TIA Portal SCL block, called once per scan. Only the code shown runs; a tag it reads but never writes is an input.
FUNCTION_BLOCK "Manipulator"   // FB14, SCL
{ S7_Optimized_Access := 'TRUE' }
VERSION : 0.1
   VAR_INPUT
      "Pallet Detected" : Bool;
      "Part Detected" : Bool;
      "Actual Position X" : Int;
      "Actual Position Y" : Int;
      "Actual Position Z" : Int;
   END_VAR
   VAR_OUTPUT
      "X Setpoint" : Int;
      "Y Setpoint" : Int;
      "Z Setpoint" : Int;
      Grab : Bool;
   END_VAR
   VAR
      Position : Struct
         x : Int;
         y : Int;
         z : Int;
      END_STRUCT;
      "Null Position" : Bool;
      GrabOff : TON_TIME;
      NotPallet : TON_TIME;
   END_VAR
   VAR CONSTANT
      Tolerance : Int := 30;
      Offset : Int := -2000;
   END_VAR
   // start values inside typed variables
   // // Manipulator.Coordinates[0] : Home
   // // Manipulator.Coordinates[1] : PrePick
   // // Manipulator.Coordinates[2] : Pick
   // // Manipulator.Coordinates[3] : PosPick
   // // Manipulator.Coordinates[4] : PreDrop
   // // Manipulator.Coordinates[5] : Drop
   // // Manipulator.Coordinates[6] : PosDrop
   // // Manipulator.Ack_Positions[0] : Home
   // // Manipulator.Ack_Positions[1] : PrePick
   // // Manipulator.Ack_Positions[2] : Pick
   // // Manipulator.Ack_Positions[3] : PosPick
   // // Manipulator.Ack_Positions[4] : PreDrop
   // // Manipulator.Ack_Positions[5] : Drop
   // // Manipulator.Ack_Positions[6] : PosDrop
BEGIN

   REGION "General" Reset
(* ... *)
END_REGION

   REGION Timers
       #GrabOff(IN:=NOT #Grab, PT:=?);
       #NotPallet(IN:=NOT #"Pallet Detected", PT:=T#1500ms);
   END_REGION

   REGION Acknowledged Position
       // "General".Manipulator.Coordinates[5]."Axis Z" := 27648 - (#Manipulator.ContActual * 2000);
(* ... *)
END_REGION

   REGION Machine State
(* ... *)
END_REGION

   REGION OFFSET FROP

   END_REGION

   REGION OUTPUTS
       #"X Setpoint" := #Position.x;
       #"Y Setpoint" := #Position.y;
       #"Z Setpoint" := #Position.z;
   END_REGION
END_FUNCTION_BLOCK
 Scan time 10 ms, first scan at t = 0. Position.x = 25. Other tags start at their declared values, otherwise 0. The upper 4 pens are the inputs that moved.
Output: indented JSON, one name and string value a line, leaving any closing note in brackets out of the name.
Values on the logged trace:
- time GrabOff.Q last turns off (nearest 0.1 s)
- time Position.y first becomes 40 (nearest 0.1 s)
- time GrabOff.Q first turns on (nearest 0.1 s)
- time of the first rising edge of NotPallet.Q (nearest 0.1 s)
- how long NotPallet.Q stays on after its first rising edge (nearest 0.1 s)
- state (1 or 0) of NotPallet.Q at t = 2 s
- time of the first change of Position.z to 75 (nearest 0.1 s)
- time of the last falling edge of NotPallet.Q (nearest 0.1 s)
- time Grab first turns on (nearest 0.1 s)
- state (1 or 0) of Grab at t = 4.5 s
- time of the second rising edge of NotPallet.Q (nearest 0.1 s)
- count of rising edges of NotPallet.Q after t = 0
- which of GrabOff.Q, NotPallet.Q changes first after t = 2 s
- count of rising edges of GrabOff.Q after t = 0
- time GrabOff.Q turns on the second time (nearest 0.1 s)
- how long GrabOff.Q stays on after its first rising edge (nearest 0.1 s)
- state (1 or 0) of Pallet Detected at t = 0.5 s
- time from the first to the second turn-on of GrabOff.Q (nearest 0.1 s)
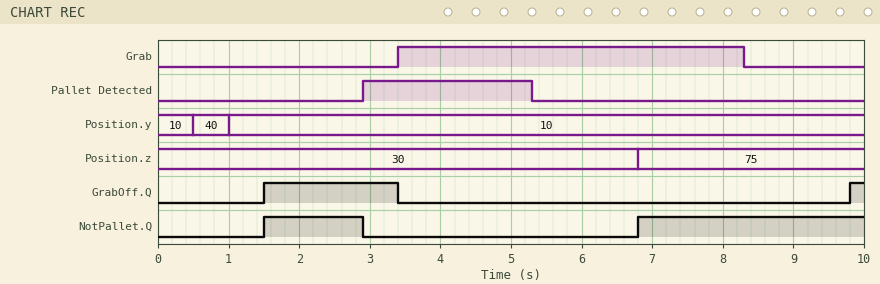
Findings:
{
  "time GrabOff.Q last turns off": "3.4 s",
  "time Position.y first becomes 40": "0.5 s",
  "time GrabOff.Q first turns on": "1.5 s",
  "time of the first rising edge of NotPallet.Q": "1.5 s",
  "how long NotPallet.Q stays on after its first rising edge": "1.4 s",
  "state (1 or 0) of NotPallet.Q at t = 2 s": "1",
  "time of the first change of Position.z to 75": "6.8 s",
  "time of the last falling edge of NotPallet.Q": "2.9 s",
  "time Grab first turns on": "3.4 s",
  "state (1 or 0) of Grab at t = 4.5 s": "1",
  "time of the second rising edge of NotPallet.Q": "6.8 s",
  "count of rising edges of NotPallet.Q after t = 0": "2",
  "which of GrabOff.Q, NotPallet.Q changes first after t = 2 s": "NotPallet.Q",
  "count of rising edges of GrabOff.Q after t = 0": "2",
  "time GrabOff.Q turns on the second time": "9.8 s",
  "how long GrabOff.Q stays on after its first rising edge": "1.9 s",
  "state (1 or 0) of Pallet Detected at t = 0.5 s": "0",
  "time from the first to the second turn-on of GrabOff.Q": "8.3 s"
}
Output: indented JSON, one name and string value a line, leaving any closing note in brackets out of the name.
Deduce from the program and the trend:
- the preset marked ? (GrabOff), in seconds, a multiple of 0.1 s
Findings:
{
  "the preset marked ? (GrabOff), in seconds, a multiple of 0.1 s": "1.5 s"
}
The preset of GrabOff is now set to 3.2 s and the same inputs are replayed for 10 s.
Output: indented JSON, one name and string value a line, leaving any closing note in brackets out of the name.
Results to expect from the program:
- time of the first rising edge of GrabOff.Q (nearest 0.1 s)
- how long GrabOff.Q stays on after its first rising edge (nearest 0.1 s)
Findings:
{
  "time of the first rising edge of GrabOff.Q": "3.2 s",
  "how long GrabOff.Q stays on after its first rising edge": "0.2 s"
}
